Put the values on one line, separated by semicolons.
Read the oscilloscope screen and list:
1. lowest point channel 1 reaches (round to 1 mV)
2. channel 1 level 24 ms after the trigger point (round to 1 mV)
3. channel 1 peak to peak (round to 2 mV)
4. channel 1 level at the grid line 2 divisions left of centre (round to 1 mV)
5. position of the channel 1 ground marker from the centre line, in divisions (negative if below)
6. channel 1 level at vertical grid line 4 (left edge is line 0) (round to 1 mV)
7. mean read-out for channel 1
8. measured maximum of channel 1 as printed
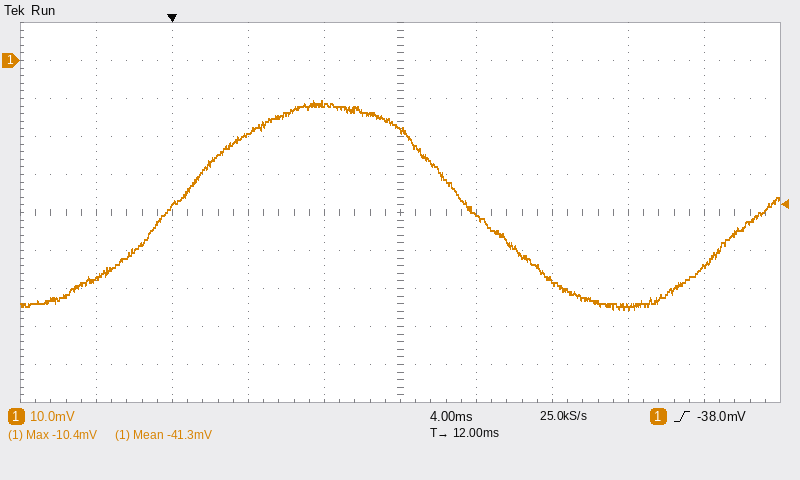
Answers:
-66 mV; -65 mV; 56 mV; -19 mV; +4.0 div; -11 mV; -41.3 mV; -10.4 mV
